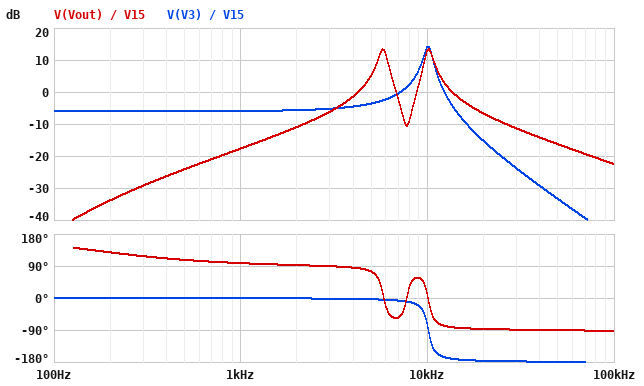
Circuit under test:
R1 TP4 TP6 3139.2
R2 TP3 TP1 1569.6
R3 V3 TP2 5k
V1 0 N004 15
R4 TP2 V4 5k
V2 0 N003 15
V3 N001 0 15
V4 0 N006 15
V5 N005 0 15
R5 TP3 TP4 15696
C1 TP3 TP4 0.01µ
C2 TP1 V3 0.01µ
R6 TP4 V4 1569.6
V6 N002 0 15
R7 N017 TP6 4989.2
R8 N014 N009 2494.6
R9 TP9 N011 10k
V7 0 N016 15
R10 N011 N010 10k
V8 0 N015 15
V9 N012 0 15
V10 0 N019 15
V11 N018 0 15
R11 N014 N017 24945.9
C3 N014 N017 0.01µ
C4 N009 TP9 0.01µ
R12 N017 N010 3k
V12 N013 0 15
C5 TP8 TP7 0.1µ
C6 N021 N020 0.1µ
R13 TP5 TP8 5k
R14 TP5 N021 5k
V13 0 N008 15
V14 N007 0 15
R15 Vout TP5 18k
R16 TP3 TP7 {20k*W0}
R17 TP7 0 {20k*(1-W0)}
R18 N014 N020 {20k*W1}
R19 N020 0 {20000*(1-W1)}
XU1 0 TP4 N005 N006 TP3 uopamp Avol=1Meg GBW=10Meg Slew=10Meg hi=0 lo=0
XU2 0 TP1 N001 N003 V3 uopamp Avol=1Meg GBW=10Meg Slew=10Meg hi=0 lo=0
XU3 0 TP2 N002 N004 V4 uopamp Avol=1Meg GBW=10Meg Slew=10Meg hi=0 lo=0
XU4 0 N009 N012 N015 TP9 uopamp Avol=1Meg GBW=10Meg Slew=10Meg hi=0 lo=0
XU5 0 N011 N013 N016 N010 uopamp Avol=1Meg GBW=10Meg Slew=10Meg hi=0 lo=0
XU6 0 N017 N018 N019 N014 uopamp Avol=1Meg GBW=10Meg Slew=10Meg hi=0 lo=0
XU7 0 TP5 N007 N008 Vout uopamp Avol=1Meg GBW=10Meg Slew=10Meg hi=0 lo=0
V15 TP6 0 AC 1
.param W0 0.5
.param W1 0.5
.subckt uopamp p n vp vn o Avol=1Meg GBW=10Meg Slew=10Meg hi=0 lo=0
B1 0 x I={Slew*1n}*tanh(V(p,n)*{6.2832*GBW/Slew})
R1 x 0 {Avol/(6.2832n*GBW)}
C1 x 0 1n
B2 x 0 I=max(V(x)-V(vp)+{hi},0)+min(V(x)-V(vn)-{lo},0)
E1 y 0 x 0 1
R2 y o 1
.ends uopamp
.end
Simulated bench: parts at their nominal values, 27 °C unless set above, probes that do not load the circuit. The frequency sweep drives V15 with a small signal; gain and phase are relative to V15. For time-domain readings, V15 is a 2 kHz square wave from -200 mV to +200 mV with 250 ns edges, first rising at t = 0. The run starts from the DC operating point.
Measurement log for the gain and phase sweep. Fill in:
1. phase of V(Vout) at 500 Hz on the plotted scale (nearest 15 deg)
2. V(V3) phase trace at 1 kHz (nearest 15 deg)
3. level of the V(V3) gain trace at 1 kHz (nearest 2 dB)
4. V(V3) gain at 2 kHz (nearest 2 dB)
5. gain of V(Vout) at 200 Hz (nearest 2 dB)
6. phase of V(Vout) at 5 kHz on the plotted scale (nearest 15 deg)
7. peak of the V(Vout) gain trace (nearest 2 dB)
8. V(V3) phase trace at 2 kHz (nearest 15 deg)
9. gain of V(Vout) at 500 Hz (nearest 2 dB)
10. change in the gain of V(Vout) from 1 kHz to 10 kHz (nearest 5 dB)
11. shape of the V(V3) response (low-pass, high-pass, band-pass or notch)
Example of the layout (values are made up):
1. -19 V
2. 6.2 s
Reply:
1. 105 deg
2. 0 deg
3. -6 dB
4. -6 dB
5. -34 dB
6. 75 deg
7. 14 dB
8. 0 deg
9. -24 dB
10. 30 dB
11. low-pass
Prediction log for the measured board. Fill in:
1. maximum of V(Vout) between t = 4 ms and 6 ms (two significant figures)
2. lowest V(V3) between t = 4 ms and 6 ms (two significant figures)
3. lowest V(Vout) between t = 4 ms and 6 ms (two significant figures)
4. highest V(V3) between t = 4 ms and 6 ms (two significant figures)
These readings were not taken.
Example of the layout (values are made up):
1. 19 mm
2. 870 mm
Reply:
1. 530 mV
2. -420 mV
3. -530 mV
4. 420 mV
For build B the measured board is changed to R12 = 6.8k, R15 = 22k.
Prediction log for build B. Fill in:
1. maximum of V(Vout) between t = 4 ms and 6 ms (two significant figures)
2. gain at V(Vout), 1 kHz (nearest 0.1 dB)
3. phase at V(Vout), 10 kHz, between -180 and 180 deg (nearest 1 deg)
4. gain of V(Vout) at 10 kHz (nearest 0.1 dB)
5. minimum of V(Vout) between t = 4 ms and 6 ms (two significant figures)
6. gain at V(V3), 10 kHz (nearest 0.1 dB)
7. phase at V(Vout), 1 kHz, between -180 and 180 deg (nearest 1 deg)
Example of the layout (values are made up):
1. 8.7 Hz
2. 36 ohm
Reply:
1. 510 mV
2. -10.4 dB
3. 11 deg
4. 14.8 dB
5. -510 mV
6. 14.2 dB
7. 97 deg
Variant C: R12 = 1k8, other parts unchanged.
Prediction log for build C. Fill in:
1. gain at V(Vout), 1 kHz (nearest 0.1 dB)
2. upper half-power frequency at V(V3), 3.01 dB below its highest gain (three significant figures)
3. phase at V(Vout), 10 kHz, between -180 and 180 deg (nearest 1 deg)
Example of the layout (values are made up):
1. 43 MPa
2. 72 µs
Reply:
1. -20.4 dB
2. 10.6 kHz
3. 7 deg
